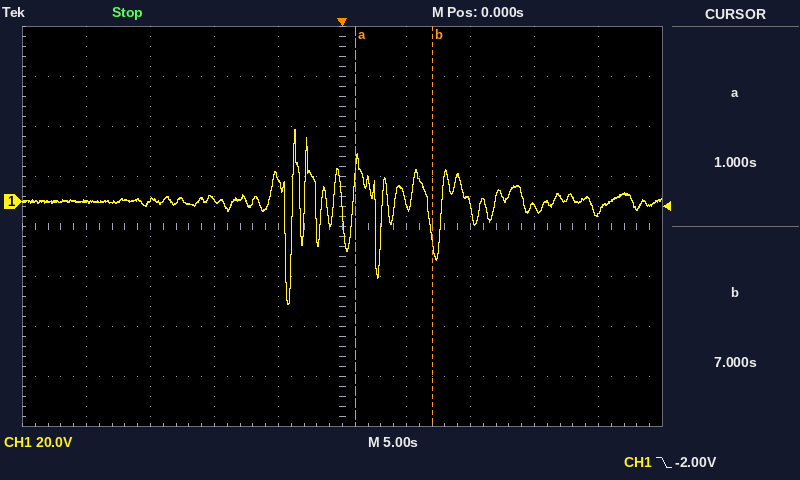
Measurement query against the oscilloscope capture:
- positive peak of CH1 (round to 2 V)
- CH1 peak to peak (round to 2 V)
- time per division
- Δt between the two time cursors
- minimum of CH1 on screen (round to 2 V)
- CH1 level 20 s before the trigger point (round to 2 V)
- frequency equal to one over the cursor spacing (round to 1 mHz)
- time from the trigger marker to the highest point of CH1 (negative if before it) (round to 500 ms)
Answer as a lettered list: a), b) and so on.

a) 28 V
b) 70 V
c) 5 s
d) 6.0 s
e) -42 V
f) 0 V
g) 167 mHz
h) -3.5 s
